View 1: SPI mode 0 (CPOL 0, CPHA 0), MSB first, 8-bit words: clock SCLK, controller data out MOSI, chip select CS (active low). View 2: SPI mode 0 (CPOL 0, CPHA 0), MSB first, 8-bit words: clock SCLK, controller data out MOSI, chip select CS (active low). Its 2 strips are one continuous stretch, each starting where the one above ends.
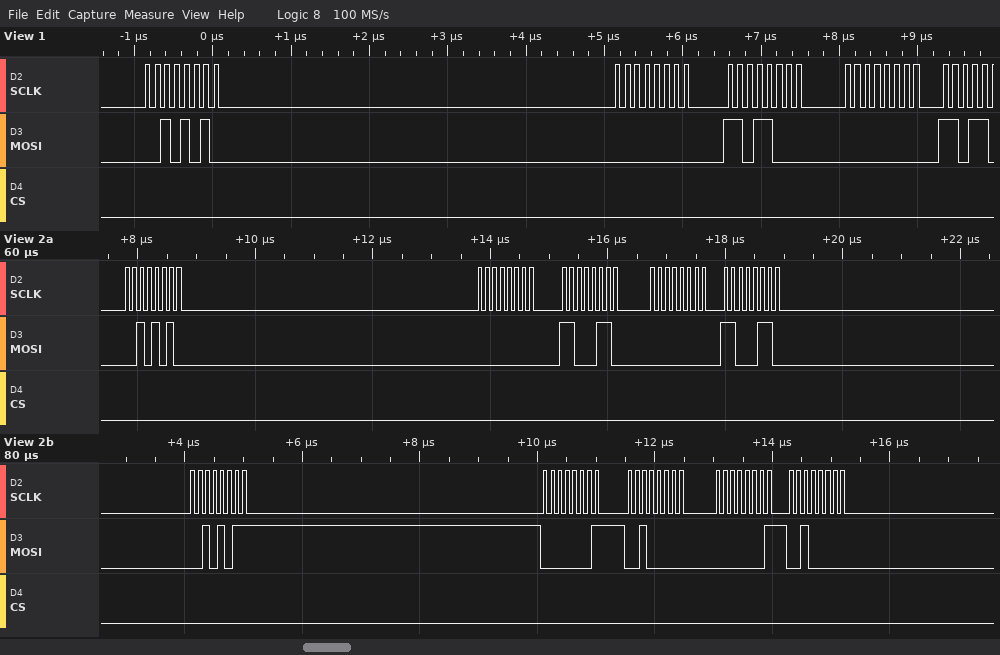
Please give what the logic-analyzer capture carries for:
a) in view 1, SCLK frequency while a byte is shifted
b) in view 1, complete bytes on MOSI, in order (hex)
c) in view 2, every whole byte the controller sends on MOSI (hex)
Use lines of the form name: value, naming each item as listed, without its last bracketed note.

in view 1, SCLK frequency while a byte is shifted: 8 MHz
in view 1, complete bytes on MOSI, in order: 2A 00 D8 00
in view 2, every whole byte the controller sends on MOSI: 2A 00 C6 00 C6 2B 01 20 01 20
